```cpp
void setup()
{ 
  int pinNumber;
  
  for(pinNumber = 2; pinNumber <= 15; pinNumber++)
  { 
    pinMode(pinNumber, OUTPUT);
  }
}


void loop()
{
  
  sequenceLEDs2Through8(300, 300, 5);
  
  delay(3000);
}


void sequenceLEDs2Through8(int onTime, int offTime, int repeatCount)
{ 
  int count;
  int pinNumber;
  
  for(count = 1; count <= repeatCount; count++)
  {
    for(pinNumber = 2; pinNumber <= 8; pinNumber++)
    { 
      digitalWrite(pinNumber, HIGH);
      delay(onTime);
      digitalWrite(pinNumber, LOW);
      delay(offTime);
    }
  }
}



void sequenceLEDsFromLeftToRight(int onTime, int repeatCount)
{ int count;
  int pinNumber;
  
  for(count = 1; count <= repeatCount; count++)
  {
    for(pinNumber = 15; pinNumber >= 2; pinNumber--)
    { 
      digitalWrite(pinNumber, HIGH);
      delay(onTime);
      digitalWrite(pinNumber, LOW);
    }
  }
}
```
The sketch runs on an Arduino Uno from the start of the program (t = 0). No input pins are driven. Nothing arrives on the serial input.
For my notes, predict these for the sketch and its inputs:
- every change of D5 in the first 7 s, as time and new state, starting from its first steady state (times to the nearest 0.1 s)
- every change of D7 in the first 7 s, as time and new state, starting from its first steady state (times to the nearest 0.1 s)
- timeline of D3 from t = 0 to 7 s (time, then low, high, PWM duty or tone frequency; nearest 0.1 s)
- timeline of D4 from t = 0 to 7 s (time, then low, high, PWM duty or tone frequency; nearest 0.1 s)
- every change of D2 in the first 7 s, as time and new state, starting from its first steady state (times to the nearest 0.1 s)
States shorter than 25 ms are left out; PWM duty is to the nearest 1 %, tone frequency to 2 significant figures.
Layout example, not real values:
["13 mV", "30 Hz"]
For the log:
["0 s low; 1.8 s high; 2.1 s low; 6 s high; 6.3 s low", "0 s low; 3 s high; 3.3 s low", "0 s low; 0.6 s high; 0.9 s low; 4.8 s high; 5.1 s low", "0 s low; 1.2 s high; 1.5 s low; 5.4 s high; 5.7 s low", "0 s high; 0.3 s low; 4.2 s high; 4.5 s low"]
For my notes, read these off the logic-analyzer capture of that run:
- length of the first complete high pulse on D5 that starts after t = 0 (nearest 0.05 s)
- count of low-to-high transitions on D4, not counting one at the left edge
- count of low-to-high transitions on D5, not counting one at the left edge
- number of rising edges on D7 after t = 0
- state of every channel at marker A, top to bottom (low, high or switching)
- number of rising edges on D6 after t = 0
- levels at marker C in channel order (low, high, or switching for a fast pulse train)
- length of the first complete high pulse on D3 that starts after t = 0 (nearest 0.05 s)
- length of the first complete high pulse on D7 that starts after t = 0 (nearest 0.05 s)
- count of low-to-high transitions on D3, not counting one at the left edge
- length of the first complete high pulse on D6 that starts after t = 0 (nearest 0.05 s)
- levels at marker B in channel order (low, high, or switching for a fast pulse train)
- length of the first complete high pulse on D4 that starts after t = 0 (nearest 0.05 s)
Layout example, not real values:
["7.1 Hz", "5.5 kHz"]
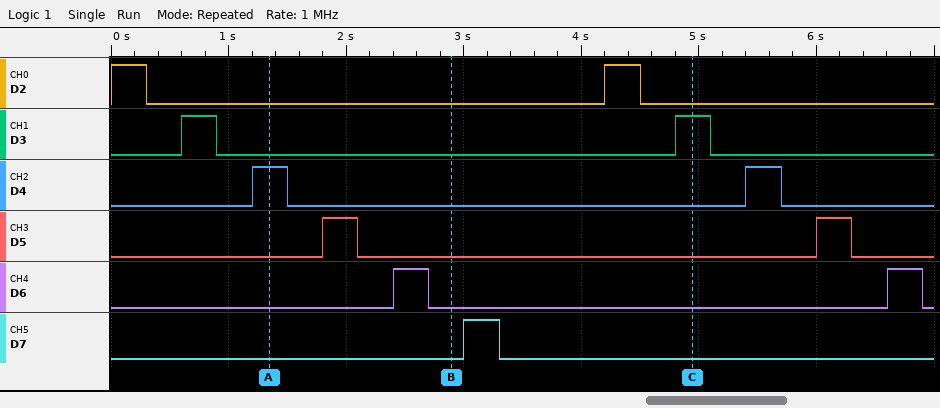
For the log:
["0.30 s", "2", "2", "1", "D2 low, D3 low, D4 high, D5 low, D6 low, D7 low", "2", "D2 low, D3 high, D4 low, D5 low, D6 low, D7 low", "0.30 s", "0.30 s", "2", "0.30 s", "D2 low, D3 low, D4 low, D5 low, D6 low, D7 low", "0.30 s"]
